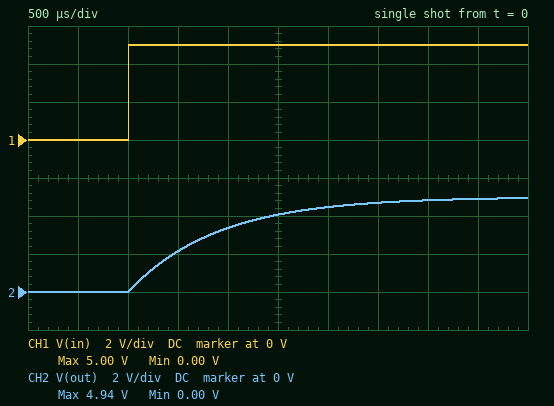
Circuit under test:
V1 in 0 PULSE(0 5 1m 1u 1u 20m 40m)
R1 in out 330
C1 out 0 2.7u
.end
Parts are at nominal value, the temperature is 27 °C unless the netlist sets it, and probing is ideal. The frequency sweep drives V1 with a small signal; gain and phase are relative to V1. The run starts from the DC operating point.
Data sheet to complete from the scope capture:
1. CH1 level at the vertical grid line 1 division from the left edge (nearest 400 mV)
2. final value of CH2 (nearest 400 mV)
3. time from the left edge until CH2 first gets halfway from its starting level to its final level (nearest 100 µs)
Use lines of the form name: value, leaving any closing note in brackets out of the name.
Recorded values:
CH1 level at the vertical grid line 1 division from the left edge: 0 V
final value of CH2: 4.8 V
time from the left edge until CH2 first gets halfway from its starting level to its final level: 1.6 ms
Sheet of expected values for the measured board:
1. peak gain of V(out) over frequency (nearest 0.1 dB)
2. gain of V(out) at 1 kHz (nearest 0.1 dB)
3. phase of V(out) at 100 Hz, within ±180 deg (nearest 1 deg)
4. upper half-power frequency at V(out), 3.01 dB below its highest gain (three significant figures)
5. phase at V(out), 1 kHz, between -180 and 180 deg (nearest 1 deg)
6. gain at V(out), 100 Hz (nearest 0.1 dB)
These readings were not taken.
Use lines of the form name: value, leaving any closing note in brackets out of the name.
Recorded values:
peak gain of V(out) over frequency: 0 dB
gain of V(out) at 1 kHz: -15.1 dB
phase of V(out) at 100 Hz, within ±180 deg: -29 deg
upper half-power frequency at V(out), 3.01 dB below its highest gain: 179 Hz
phase at V(out), 1 kHz, between -180 and 180 deg: -80 deg
gain at V(out), 100 Hz: -1.2 dB
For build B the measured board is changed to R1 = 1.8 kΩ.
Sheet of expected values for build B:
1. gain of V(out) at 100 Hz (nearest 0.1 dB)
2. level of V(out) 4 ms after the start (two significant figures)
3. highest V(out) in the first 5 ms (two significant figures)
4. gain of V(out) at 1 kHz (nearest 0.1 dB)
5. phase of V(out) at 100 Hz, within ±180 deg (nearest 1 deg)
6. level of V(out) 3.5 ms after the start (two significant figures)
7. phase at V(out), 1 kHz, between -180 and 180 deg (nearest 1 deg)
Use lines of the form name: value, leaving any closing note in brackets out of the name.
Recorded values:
gain of V(out) at 100 Hz: -10.1 dB
level of V(out) 4 ms after the start: 2.3 V
highest V(out) in the first 5 ms: 2.8 V
gain of V(out) at 1 kHz: -29.7 dB
phase of V(out) at 100 Hz, within ±180 deg: -72 deg
level of V(out) 3.5 ms after the start: 2.0 V
phase at V(out), 1 kHz, between -180 and 180 deg: -88 deg
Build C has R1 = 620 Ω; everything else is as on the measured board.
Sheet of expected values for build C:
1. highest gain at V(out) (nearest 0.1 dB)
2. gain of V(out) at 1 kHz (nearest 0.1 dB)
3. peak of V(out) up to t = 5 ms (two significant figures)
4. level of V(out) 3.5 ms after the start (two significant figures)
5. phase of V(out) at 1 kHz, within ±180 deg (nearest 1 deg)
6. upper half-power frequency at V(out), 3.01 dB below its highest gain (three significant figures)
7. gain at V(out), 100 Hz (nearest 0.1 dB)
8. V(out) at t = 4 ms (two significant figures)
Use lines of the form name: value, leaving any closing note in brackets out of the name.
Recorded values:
highest gain at V(out): 0 dB
gain of V(out) at 1 kHz: -20.5 dB
peak of V(out) up to t = 5 ms: 4.5 V
level of V(out) 3.5 ms after the start: 3.9 V
phase of V(out) at 1 kHz, within ±180 deg: -85 deg
upper half-power frequency at V(out), 3.01 dB below its highest gain: 95.1 Hz
gain at V(out), 100 Hz: -3.2 dB
V(out) at t = 4 ms: 4.2 V
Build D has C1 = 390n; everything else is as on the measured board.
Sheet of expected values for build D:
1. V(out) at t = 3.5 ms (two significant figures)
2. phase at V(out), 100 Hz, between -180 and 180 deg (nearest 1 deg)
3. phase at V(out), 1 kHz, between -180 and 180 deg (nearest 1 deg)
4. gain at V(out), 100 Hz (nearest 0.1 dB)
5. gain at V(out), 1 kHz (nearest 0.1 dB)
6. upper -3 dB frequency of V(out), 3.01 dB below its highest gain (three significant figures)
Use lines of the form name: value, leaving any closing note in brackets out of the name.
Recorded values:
V(out) at t = 3.5 ms: 5.0 V
phase at V(out), 100 Hz, between -180 and 180 deg: -5 deg
phase at V(out), 1 kHz, between -180 and 180 deg: -39 deg
gain at V(out), 100 Hz: 0 dB
gain at V(out), 1 kHz: -2.2 dB
upper -3 dB frequency of V(out), 3.01 dB below its highest gain: 1.24 kHz
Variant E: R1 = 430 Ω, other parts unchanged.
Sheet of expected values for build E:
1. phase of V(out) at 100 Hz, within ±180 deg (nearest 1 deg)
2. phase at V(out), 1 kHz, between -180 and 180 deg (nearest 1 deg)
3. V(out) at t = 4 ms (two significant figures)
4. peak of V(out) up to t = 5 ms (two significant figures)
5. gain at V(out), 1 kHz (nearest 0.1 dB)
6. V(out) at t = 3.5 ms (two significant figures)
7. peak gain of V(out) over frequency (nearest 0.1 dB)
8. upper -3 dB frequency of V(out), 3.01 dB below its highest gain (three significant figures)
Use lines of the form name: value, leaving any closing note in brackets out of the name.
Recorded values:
phase of V(out) at 100 Hz, within ±180 deg: -36 deg
phase at V(out), 1 kHz, between -180 and 180 deg: -82 deg
V(out) at t = 4 ms: 4.6 V
peak of V(out) up to t = 5 ms: 4.8 V
gain at V(out), 1 kHz: -17.3 dB
V(out) at t = 3.5 ms: 4.4 V
peak gain of V(out) over frequency: 0 dB
upper -3 dB frequency of V(out), 3.01 dB below its highest gain: 137 Hz
